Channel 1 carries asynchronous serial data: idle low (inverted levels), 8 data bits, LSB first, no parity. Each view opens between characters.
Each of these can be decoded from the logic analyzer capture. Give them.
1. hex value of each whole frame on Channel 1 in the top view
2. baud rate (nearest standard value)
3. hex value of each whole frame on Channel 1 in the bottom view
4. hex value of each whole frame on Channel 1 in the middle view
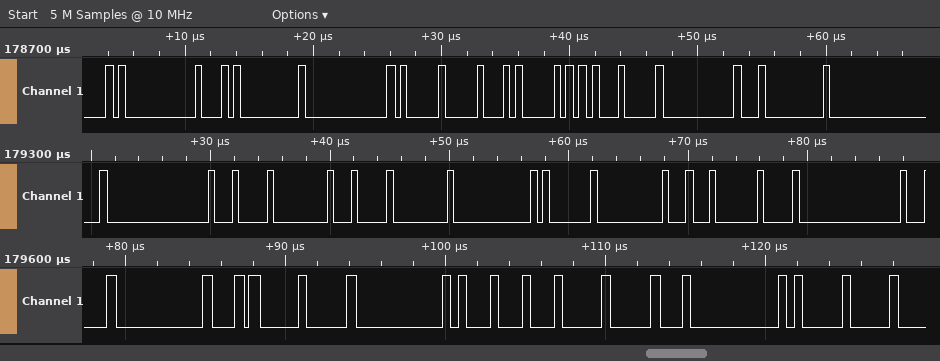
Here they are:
FD, D7, FF, 7D, D7, D5, DF, F7, FF
2000000 baud
FF, D7, DF, DD, F7, DF, FF, 7D
FF, F7, FF, F7, FF, FF, FD, FF, 77, DF
